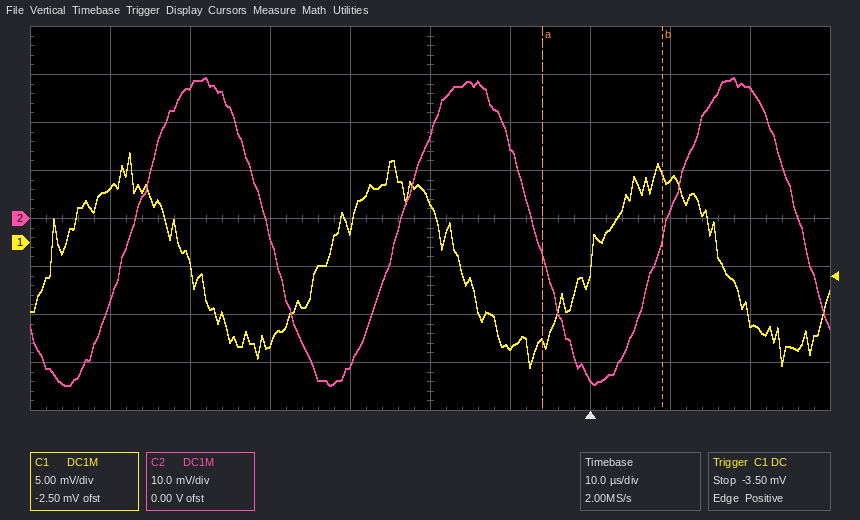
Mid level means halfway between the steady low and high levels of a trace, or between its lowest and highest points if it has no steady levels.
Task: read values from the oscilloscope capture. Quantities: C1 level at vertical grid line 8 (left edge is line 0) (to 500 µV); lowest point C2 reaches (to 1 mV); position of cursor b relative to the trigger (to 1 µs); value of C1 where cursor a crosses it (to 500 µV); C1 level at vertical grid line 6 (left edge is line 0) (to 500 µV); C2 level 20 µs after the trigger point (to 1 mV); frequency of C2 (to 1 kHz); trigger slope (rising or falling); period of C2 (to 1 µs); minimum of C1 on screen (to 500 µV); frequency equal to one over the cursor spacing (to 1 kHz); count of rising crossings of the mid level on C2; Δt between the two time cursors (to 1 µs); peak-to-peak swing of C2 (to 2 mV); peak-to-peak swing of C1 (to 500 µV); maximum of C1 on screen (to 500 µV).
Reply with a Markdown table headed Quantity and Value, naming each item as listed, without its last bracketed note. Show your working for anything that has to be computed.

| Quantity | Value |
|---|---|
| C1 level at vertical grid line 8 (left edge is line 0) | 6.5 mV |
| lowest point C2 reaches | -35 mV |
| position of cursor b relative to the trigger | +9 µs |
| value of C1 where cursor a crosses it | -10.5 mV |
| C1 level at vertical grid line 6 (left edge is line 0) | -11.0 mV |
| C2 level 20 µs after the trigger point | 27 mV |
| frequency of C2 | 1 / 33 µs ≈ 30 kHz |
| trigger slope | rising |
| period of C2 | 33 µs |
| minimum of C1 on screen | -13.0 mV |
| frequency equal to one over the cursor spacing | 1 / 15 µs ≈ 67 kHz |
| count of rising crossings of the mid level on C2 | 3 |
| Δt between the two time cursors | 15 µs |
| peak-to-peak swing of C2 | 64 mV |
| peak-to-peak swing of C1 | 9.5 mV − (-13.0 mV) = 22.5 mV |
| maximum of C1 on screen | 9.5 mV |
